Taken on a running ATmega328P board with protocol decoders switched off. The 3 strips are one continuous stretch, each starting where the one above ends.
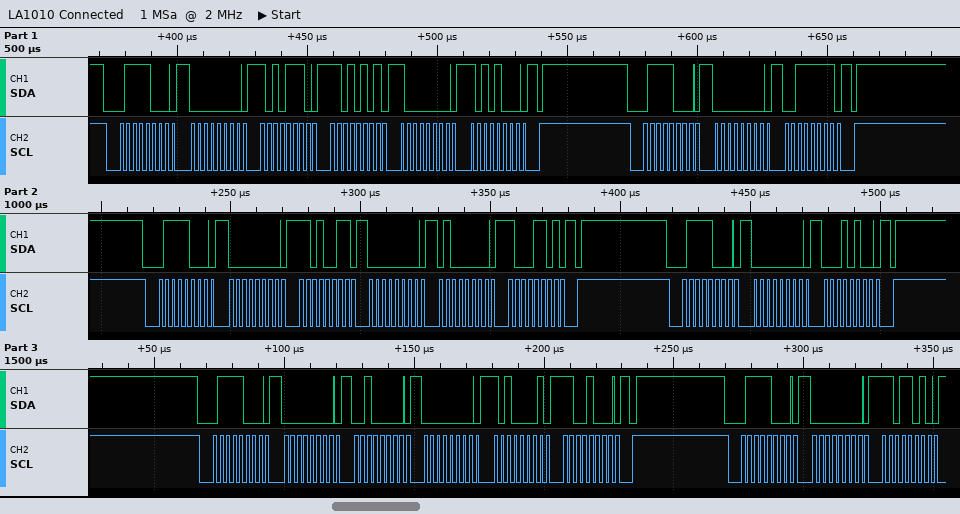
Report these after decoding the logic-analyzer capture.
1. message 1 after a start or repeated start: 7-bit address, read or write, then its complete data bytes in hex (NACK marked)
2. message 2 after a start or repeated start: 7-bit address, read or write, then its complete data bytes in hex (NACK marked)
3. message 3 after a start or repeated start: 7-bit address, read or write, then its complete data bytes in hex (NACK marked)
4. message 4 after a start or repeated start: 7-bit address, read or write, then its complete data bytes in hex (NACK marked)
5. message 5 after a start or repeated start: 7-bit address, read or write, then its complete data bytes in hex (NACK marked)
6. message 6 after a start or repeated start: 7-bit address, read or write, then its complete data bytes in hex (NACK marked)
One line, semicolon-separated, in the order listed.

0x3C write: 00 AE D5 80 A8; 0x3C write: 00 3F; 0x3C write: 00 D3 00 40 8D; 0x3C write: 00 14; 0x3C write: 00 20 00 A1 C8; 0x3C write: 00 DA
